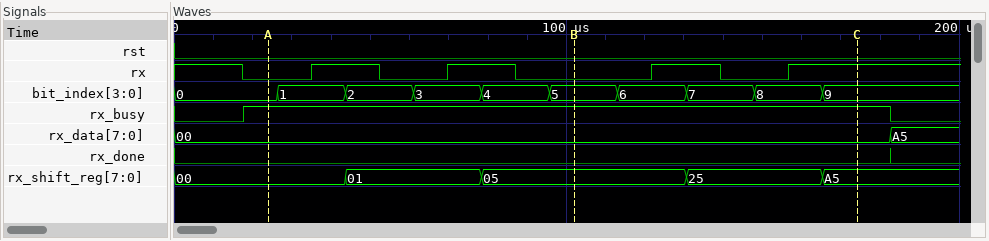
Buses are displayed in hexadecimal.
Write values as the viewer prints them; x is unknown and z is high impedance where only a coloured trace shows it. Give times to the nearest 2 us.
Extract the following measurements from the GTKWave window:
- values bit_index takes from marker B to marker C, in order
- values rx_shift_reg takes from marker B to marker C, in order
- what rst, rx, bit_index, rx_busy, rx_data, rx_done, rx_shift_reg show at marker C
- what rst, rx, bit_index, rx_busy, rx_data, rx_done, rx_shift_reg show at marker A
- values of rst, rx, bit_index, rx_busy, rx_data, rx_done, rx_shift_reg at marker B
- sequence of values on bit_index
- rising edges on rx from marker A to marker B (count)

5, 6, 7, 8, 9
05, 25, A5
rst=0, rx=1, bit_index=9, rx_busy=1, rx_data=00, rx_done=0, rx_shift_reg=A5
rst=0, rx=0, bit_index=0, rx_busy=1, rx_data=00, rx_done=0, rx_shift_reg=00
rst=0, rx=0, bit_index=5, rx_busy=1, rx_data=00, rx_done=0, rx_shift_reg=05
0, 1, 2, 3, 4, 5, 6, 7, 8, 9
2
